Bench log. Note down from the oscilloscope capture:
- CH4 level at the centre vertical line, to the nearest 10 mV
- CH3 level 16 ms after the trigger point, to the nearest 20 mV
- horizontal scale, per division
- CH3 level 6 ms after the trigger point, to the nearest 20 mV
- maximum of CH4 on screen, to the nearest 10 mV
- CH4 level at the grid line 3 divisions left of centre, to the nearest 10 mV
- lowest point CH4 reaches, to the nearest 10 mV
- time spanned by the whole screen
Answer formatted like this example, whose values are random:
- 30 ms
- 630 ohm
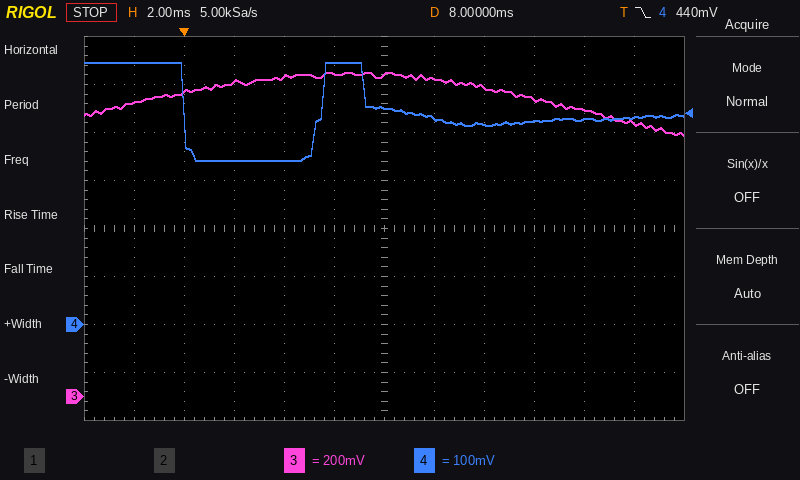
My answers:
- 450 mV
- 1.20 V
- 2 ms
- 1.34 V
- 550 mV
- 340 mV
- 340 mV
- 24 ms
